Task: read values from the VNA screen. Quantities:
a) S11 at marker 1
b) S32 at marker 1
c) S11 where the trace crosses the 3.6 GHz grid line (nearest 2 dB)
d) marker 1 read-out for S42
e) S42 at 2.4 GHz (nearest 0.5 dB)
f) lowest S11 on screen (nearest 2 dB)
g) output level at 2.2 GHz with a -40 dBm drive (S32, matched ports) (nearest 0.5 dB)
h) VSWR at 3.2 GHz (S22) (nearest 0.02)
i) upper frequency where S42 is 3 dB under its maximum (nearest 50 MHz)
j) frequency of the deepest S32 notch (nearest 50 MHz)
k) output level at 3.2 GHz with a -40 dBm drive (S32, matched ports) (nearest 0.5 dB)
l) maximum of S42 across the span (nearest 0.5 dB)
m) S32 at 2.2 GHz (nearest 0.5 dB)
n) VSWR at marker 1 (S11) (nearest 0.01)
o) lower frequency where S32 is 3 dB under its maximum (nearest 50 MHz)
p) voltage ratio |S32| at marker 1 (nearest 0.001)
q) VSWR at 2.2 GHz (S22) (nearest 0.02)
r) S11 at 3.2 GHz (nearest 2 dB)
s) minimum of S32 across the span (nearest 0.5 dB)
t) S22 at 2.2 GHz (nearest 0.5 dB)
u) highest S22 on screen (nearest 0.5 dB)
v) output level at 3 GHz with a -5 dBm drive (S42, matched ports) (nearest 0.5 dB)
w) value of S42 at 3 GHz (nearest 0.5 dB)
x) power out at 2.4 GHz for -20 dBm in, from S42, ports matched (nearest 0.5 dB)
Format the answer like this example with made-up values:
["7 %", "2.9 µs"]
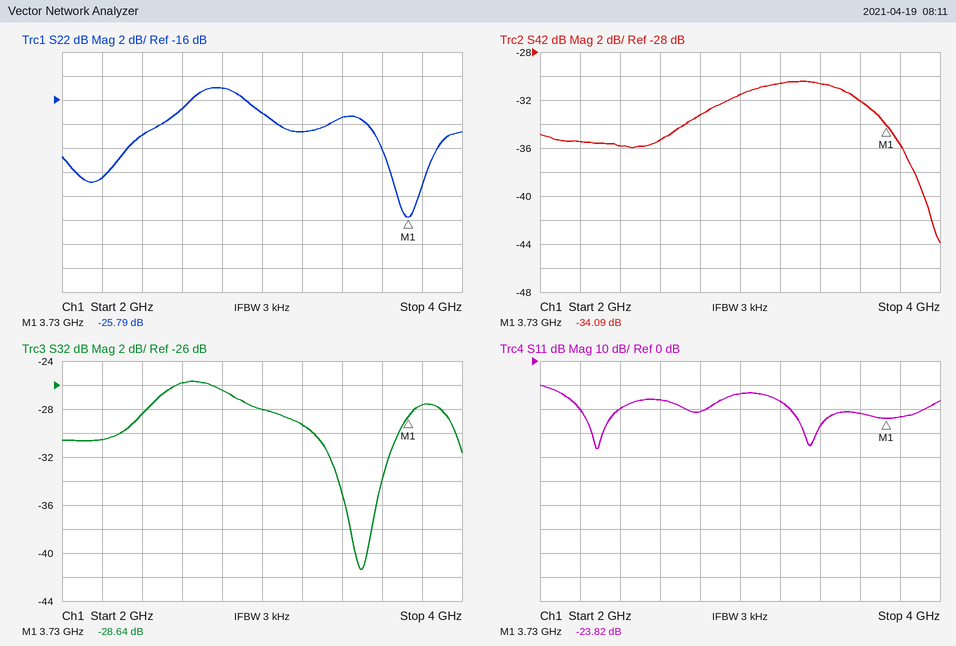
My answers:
["-23.82 dB", "-28.64 dB", "-22 dB", "-34.09 dB", "-36.0 dB", "-36 dB", "-70.5 dBm", "1.26", "3.70 GHz", "3.50 GHz", "-69.5 dBm", "-30.5 dB", "-30.5 dB", "1.14", "2.40 GHz", "0.037", "1.16", "-16 dB", "-41.5 dB", "-22.5 dB", "-15.0 dB", "-36.5 dBm", "-31.5 dB", "-56.0 dBm"]
